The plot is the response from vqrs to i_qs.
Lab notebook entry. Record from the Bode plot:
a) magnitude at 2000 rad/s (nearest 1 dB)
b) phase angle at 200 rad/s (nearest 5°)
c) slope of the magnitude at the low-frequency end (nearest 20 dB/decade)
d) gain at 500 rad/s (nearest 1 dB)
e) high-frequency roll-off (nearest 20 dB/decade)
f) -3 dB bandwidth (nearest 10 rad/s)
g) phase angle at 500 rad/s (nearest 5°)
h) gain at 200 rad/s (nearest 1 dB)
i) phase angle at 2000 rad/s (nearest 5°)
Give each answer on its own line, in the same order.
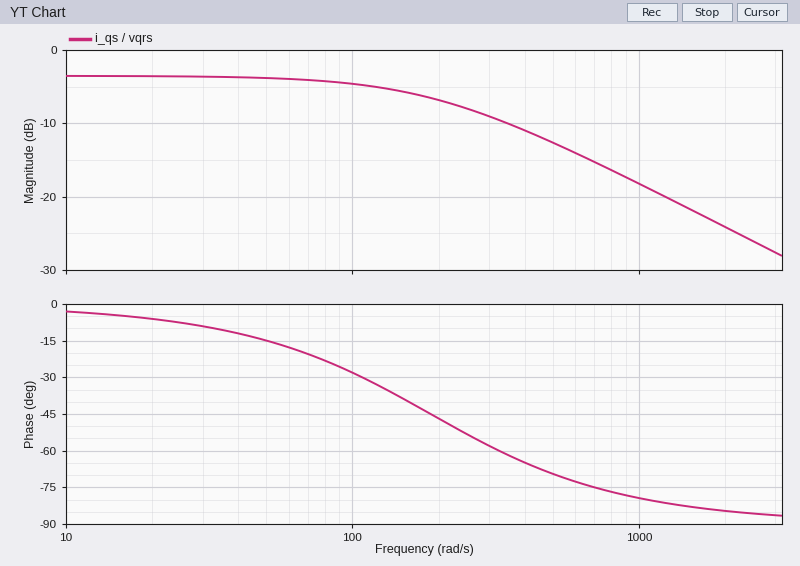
-24 dB
-45°
0 dB/decade
-13 dB
-20 dB/decade
190 rad/s
-70°
-7 dB
-85°
